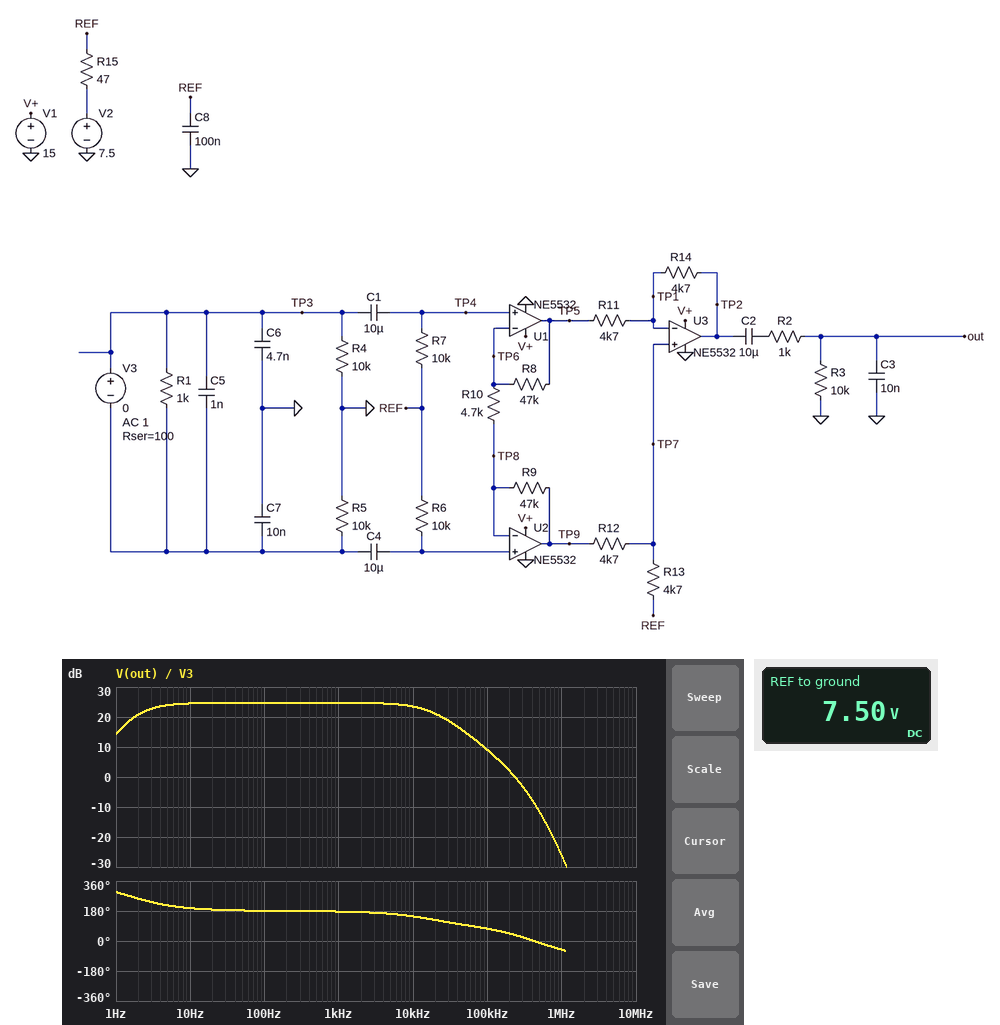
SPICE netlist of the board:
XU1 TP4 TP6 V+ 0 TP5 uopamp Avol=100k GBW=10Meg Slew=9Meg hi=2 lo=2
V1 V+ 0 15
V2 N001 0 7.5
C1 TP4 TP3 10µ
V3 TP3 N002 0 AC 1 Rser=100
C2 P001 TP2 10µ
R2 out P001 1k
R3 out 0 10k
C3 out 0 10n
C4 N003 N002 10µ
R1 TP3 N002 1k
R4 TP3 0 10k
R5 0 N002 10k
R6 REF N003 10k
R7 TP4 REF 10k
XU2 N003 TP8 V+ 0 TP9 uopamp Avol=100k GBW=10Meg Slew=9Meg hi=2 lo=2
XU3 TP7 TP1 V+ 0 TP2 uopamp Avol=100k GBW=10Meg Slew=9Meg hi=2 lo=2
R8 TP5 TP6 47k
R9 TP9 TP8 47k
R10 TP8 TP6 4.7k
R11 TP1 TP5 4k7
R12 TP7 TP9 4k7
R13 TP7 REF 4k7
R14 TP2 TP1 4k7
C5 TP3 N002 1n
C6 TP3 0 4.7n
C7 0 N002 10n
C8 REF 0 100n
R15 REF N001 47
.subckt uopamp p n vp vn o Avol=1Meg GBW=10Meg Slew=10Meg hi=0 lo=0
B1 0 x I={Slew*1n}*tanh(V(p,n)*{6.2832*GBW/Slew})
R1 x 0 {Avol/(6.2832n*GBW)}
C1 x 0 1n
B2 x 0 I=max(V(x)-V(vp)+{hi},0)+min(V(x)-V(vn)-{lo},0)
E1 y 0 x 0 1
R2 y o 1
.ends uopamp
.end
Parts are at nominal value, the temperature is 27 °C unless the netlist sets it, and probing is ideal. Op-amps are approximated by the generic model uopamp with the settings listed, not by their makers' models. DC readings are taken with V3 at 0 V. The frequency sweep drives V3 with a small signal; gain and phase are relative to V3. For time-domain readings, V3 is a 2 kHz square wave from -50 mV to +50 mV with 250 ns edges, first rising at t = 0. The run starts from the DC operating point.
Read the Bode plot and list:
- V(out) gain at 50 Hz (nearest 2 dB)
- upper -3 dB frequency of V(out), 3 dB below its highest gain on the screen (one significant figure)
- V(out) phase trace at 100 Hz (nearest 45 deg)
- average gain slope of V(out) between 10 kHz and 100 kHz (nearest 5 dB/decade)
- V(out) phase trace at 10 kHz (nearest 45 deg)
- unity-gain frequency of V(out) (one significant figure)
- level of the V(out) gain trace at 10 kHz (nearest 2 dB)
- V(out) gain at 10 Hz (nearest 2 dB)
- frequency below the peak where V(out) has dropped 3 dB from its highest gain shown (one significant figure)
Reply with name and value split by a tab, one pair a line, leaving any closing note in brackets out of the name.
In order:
V(out) gain at 50 Hz	24 dB
upper -3 dB frequency of V(out), 3 dB below its highest gain on the screen	20 kHz
V(out) phase trace at 100 Hz	180 deg
average gain slope of V(out) between 10 kHz and 100 kHz	-15 dB/decade
V(out) phase trace at 10 kHz	135 deg
unity-gain frequency of V(out)	200 kHz
level of the V(out) gain trace at 10 kHz	24 dB
V(out) gain at 10 Hz	24 dB
frequency below the peak where V(out) has dropped 3 dB from its highest gain shown	2 Hz
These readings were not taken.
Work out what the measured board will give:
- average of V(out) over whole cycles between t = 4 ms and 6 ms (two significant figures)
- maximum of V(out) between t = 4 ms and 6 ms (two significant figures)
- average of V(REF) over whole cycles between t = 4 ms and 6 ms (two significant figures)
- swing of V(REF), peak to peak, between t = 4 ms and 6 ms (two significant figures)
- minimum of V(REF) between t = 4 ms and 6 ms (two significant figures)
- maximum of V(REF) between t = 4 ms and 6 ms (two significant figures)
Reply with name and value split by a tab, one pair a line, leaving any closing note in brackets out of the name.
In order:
average of V(out) over whole cycles between t = 4 ms and 6 ms	-780 mV
maximum of V(out) between t = 4 ms and 6 ms	94 mV
average of V(REF) over whole cycles between t = 4 ms and 6 ms	7.5 V
swing of V(REF), peak to peak, between t = 4 ms and 6 ms	4.7 mV
minimum of V(REF) between t = 4 ms and 6 ms	7.5 V
maximum of V(REF) between t = 4 ms and 6 ms	7.5 V
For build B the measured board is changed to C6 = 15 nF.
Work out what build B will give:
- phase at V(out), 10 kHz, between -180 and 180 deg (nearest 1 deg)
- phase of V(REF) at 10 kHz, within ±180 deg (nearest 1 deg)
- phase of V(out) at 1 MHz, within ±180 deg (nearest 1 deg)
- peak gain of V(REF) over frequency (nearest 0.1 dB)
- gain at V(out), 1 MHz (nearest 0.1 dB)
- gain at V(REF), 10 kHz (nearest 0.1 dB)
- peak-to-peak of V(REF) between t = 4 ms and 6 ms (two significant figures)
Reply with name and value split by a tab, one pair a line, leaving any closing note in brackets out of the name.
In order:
phase at V(out), 10 kHz, between -180 and 180 deg	147 deg
phase of V(REF) at 10 kHz, within ±180 deg	161 deg
phase of V(out) at 1 MHz, within ±180 deg	-61 deg
peak gain of V(REF) over frequency	-26.5 dB
gain at V(out), 1 MHz	-30.2 dB
gain at V(REF), 10 kHz	-26.8 dB
peak-to-peak of V(REF) between t = 4 ms and 6 ms	4.8 mV
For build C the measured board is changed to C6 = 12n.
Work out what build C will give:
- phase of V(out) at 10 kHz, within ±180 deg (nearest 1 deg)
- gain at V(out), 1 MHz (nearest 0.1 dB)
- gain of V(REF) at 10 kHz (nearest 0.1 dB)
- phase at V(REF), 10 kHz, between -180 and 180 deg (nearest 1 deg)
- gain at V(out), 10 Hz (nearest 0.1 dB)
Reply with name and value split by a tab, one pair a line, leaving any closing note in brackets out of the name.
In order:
phase of V(out) at 10 kHz, within ±180 deg	147 deg
gain at V(out), 1 MHz	-29.5 dB
gain of V(REF) at 10 kHz	-26.9 dB
phase at V(REF), 10 kHz, between -180 and 180 deg	161 deg
gain at V(out), 10 Hz	24.5 dB
